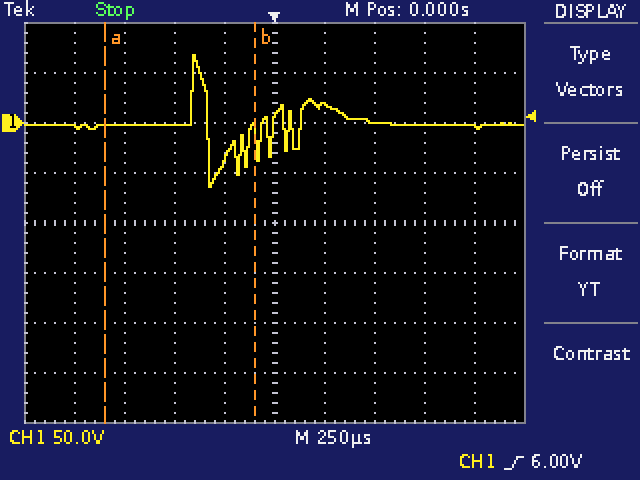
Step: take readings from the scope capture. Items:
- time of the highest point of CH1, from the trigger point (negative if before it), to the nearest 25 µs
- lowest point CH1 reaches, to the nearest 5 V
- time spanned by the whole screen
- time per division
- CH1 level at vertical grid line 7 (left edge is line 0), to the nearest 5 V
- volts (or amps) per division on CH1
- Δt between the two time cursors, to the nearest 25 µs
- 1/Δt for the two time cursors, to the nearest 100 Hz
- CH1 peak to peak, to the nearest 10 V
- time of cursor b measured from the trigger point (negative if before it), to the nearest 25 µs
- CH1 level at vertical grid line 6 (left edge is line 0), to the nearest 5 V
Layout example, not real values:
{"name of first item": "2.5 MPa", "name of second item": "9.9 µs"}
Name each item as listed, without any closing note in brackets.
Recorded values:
{"time of the highest point of CH1, from the trigger point (negative if before it), to the nearest 25 µs": "-400 µs", "lowest point CH1 reaches, to the nearest 5 V": "-65 V", "time spanned by the whole screen": "2.5 ms", "time per division": "250 µs", "CH1 level at vertical grid line 7 (left edge is line 0), to the nearest 5 V": "0 V", "volts (or amps) per division on CH1": "50 V", "Δt between the two time cursors, to the nearest 25 µs": "750 µs", "1/Δt for the two time cursors, to the nearest 100 Hz": "1.3 kHz", "CH1 peak to peak, to the nearest 10 V": "130 V", "time of cursor b measured from the trigger point (negative if before it), to the nearest 25 µs": "-100 µs", "CH1 level at vertical grid line 6 (left edge is line 0), to the nearest 5 V": "20 V"}
